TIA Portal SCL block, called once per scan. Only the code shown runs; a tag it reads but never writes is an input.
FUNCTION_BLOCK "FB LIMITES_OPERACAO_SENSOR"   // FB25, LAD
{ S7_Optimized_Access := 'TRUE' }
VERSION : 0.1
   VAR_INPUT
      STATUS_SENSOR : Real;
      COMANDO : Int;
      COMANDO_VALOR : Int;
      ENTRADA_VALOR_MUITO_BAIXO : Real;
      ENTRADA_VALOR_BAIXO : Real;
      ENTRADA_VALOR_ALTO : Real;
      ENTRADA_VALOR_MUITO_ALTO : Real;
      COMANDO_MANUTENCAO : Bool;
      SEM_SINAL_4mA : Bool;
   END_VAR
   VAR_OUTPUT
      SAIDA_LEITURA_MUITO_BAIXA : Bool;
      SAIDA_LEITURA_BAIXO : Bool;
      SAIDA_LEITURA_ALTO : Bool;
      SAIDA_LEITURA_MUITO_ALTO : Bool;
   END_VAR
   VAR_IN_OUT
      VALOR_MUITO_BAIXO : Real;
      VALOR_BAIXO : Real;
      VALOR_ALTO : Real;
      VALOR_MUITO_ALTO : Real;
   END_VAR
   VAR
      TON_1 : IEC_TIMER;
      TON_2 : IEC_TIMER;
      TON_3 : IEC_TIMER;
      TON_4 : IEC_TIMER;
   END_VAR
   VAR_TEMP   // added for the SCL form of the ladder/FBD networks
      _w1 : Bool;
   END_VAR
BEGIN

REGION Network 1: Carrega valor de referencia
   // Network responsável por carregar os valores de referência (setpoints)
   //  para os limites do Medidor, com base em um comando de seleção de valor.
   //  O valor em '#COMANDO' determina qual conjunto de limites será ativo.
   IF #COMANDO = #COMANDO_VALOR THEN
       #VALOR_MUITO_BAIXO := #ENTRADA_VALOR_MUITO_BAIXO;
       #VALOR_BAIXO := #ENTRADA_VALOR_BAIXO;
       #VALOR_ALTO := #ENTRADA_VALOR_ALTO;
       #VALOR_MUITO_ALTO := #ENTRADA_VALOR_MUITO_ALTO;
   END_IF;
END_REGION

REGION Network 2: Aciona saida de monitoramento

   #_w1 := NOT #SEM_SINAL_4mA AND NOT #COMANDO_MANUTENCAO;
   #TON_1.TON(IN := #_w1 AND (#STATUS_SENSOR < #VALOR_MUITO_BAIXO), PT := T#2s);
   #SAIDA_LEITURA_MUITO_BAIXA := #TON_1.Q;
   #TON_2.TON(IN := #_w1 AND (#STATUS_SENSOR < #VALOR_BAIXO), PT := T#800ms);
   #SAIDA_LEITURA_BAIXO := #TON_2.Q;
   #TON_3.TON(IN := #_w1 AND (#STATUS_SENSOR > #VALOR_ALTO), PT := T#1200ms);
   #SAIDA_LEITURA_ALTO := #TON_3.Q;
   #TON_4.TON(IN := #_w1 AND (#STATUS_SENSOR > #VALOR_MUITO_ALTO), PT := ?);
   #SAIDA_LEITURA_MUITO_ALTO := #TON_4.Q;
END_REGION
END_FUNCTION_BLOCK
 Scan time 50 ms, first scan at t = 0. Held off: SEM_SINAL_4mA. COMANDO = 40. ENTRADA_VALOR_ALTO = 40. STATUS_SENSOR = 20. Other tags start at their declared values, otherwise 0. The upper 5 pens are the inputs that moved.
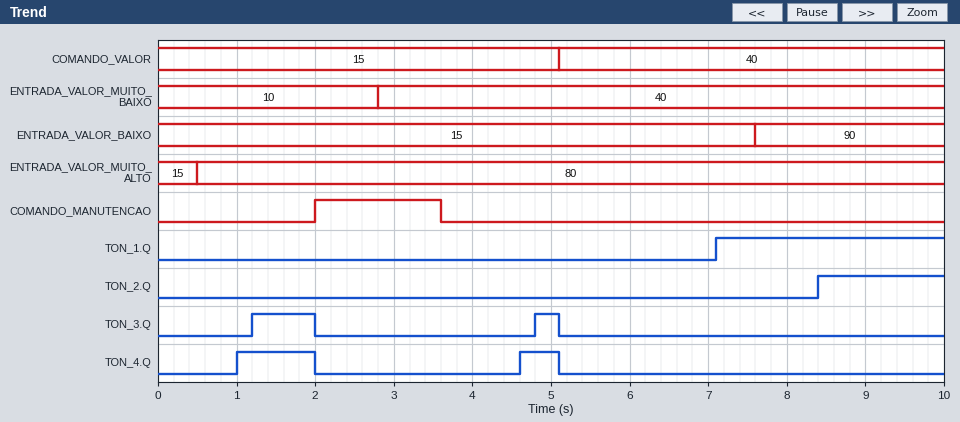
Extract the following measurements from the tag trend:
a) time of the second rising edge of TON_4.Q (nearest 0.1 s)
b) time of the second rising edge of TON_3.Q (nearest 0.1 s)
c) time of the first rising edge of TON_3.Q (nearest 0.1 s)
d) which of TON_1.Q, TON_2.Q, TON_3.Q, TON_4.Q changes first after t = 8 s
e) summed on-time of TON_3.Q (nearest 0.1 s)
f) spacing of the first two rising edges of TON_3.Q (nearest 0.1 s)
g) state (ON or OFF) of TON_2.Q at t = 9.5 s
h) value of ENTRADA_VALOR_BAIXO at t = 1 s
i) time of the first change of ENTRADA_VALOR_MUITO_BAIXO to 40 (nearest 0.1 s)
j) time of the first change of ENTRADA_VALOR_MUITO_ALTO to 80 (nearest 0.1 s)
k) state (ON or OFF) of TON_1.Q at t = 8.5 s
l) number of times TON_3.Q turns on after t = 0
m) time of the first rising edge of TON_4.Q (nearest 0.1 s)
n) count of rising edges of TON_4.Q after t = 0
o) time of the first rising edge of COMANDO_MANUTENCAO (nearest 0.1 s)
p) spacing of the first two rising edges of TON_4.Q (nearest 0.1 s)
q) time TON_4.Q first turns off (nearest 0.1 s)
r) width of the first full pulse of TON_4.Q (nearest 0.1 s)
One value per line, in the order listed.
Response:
4.6 s
4.8 s
1.2 s
TON_2.Q
1.1 s
3.6 s
ON
15
2.8 s
0.5 s
ON
2
1.0 s
2
2.0 s
3.6 s
2.0 s
1.0 s
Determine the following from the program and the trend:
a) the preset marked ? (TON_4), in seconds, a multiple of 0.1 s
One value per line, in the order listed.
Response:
1.0 s
